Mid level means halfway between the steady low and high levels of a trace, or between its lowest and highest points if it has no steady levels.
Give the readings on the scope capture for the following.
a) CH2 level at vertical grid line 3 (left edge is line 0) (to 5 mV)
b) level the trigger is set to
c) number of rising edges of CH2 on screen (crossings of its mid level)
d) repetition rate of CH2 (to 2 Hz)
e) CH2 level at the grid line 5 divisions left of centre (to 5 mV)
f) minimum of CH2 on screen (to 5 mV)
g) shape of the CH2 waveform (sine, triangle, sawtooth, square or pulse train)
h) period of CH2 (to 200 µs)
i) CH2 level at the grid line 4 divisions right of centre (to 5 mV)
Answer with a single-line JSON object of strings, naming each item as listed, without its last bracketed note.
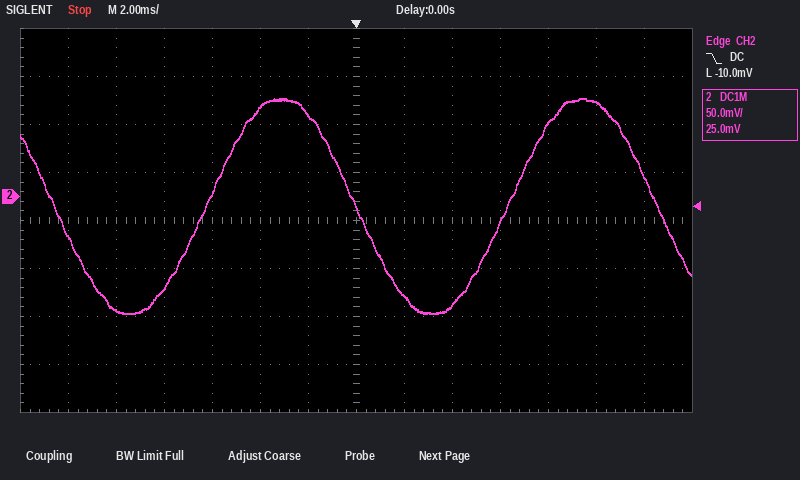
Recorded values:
{"CH2 level at vertical grid line 3 (left edge is line 0)": "-95 mV", "level the trigger is set to": "-10.0 mV", "number of rising edges of CH2 on screen": "2", "repetition rate of CH2": "80 Hz", "CH2 level at the grid line 5 divisions left of centre": "-120 mV", "minimum of CH2 on screen": "-120 mV", "shape of the CH2 waveform": "sine", "period of CH2": "12.6 ms", "CH2 level at the grid line 4 divisions right of centre": "75 mV"}
